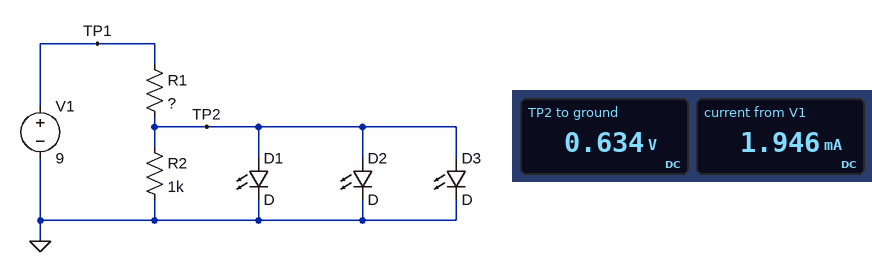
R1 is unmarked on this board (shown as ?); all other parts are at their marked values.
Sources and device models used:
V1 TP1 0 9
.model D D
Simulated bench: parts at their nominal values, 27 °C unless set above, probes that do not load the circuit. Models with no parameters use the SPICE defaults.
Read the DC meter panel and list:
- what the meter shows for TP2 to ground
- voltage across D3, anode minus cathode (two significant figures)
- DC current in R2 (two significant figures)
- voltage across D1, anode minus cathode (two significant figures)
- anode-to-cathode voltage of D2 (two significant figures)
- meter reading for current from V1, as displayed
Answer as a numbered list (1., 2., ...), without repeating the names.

1. 0.634 V
2. 630 mV
3. 630 µA
4. 630 mV
5. 630 mV
6. 1.946 mA
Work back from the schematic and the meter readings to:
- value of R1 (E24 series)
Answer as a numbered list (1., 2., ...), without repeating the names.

1. 4.3 kΩ
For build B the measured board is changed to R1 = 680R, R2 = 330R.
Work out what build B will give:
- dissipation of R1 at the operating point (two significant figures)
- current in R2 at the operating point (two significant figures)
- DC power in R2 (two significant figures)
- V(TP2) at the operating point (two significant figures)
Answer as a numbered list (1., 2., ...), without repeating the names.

1. 100 mW
2. 2.1 mA
3. 1.4 mW
4. 690 mV
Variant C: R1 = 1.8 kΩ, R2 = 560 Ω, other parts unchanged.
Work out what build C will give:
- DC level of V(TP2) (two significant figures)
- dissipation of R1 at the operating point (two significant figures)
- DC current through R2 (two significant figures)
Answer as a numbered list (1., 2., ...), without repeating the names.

1. 660 mV
2. 39 mW
3. 1.2 mA
